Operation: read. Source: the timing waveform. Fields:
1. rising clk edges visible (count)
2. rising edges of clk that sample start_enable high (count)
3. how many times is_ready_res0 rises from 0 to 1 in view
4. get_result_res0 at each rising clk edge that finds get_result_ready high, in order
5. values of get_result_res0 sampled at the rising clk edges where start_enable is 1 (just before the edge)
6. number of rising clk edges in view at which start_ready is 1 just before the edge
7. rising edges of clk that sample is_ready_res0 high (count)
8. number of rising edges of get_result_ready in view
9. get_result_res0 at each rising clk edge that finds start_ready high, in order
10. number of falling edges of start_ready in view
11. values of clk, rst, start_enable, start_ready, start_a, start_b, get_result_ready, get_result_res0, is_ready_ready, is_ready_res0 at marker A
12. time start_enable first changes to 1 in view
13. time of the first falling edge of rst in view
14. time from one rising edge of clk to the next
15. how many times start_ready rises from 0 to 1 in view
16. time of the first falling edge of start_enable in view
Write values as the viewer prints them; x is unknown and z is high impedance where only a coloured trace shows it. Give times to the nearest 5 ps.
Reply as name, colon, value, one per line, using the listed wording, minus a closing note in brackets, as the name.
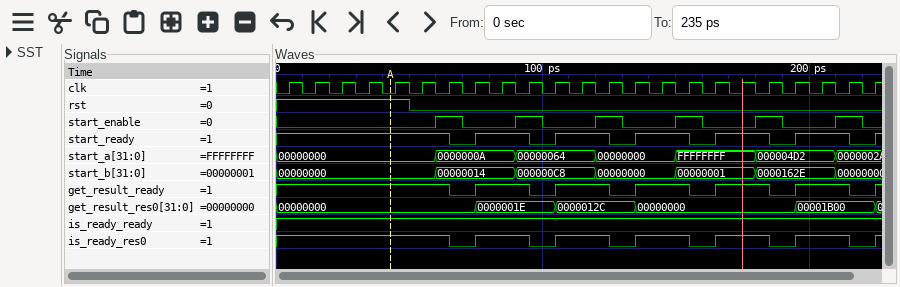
rising clk edges visible: 23
rising edges of clk that sample start_enable high: 6
how many times is_ready_res0 rises from 0 to 1 in view: 6
get_result_res0 at each rising clk edge that finds get_result_ready high, in order: 00000000, 00000000, 00000000, 00000000, 00000000, 00000000, 00000000, 0000001E, 0000001E, 0000012C, 0000012C, 00000000, 00000000, 00000000, 00000000, 00001B00, 00001B00
values of get_result_res0 sampled at the rising clk edges where start_enable is 1: 00000000, 0000001E, 0000012C, 00000000, 00000000, 00001B00
number of rising clk edges in view at which start_ready is 1 just before the edge: 17
rising edges of clk that sample is_ready_res0 high: 17
number of rising edges of get_result_ready in view: 6
get_result_res0 at each rising clk edge that finds start_ready high, in order: 00000000, 00000000, 00000000, 00000000, 00000000, 00000000, 00000000, 0000001E, 0000001E, 0000012C, 0000012C, 00000000, 00000000, 00000000, 00000000, 00001B00, 00001B00
number of falling edges of start_ready in view: 6
values of clk, rst, start_enable, start_ready, start_a, start_b, get_result_ready, get_result_res0, is_ready_ready, is_ready_res0 at marker A: clk=0, rst=1, start_enable=0, start_ready=1, start_a=00000000, start_b=00000000, get_result_ready=1, get_result_res0=00000000, is_ready_ready=1, is_ready_res0=1
time start_enable first changes to 1 in view: 60 ps
time of the first falling edge of rst in view: 50 ps
time from one rising edge of clk to the next: 10 ps
how many times start_ready rises from 0 to 1 in view: 6
time of the first falling edge of start_enable in view: 70 ps
